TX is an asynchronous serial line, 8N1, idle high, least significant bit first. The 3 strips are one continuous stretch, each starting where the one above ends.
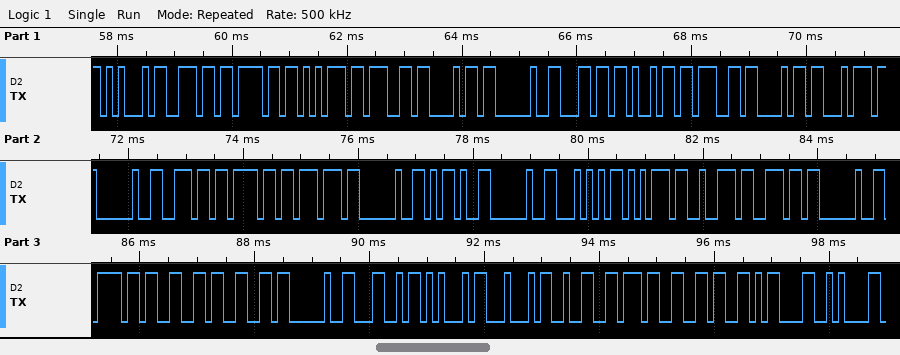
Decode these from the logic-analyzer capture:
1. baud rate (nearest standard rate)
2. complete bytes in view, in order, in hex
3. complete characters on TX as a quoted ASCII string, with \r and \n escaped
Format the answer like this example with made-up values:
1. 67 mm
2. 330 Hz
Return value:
1. 9600 baud
2. 45 6E 6F 75 67 68 20 6C 69 67 68 74 20 6E 6F 77 20 2D 20 54 75 72 6E 20 6F 66 66 20 4C 45 44 32 37 36 0D 0A
3. "Enough light now - Turn off LED276\r\n"
